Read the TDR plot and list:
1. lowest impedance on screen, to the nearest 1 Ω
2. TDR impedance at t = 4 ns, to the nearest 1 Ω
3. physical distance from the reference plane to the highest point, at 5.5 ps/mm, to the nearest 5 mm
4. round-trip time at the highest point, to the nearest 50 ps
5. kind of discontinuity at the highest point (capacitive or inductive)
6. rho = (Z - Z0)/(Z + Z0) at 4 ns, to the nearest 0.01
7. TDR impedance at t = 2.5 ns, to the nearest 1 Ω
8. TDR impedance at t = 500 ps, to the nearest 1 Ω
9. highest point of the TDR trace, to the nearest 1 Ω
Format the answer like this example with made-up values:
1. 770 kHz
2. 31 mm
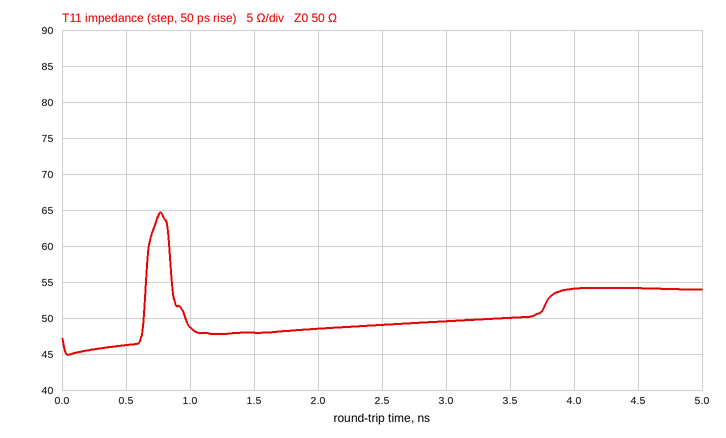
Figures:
1. 45 Ω
2. 54 Ω
3. 70 mm
4. 750 ps
5. inductive
6. +0.04
7. 49 Ω
8. 46 Ω
9. 65 Ω
